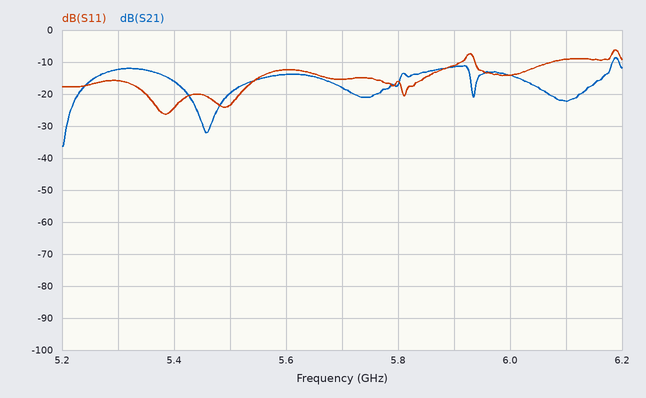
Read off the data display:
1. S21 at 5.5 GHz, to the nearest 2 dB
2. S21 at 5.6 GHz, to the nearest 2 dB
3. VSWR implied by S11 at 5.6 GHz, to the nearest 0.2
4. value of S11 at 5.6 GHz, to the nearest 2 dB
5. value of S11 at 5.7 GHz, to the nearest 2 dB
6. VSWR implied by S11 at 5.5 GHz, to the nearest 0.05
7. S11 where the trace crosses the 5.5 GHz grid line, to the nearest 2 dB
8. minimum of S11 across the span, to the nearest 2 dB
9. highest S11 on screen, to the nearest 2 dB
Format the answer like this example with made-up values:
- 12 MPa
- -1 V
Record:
- -20 dB
- -14 dB
- 1.6
- -12 dB
- -16 dB
- 1.15
- -24 dB
- -26 dB
- -6 dB
